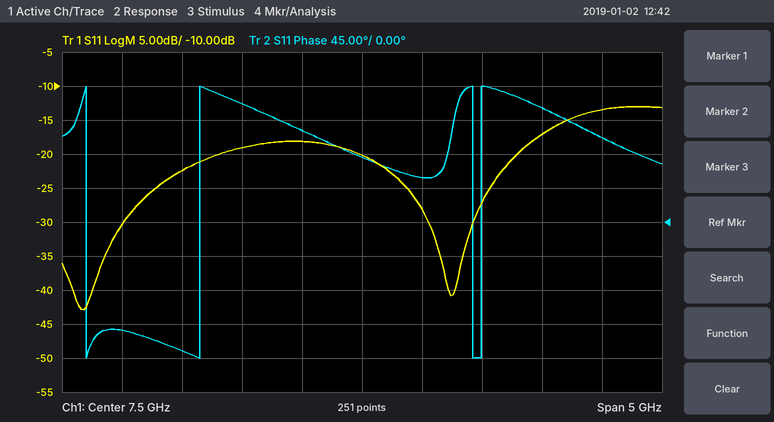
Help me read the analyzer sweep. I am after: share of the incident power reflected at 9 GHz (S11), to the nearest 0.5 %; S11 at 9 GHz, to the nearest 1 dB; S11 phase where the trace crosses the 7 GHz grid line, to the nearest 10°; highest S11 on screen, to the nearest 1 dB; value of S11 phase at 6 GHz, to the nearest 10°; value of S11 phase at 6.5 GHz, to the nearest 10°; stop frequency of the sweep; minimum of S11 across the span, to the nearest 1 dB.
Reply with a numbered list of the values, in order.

1. 2.0 %
2. -17 dB
3. 120°
4. -13 dB
5. -170°
6. 160°
7. 10 GHz
8. -43 dB
